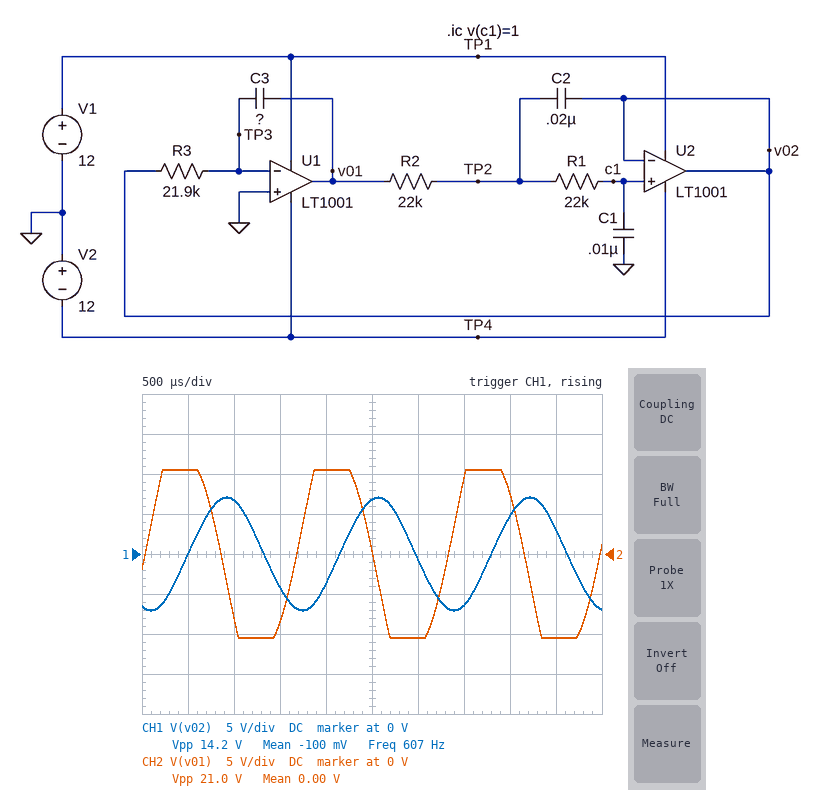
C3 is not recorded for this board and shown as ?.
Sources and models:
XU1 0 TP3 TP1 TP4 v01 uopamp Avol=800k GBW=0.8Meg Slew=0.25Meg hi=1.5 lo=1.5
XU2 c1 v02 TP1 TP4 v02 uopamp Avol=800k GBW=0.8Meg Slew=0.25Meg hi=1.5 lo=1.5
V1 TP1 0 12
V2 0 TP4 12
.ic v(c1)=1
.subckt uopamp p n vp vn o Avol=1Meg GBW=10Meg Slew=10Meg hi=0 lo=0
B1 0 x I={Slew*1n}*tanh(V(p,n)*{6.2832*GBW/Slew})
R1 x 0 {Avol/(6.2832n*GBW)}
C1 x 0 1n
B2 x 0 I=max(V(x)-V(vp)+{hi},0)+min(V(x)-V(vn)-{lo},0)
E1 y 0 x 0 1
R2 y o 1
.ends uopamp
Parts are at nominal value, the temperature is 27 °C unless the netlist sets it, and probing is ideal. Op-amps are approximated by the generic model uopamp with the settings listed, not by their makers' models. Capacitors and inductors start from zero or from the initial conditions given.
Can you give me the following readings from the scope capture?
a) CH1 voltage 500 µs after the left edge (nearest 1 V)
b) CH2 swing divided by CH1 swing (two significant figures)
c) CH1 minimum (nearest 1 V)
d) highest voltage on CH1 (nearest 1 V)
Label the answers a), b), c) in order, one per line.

a) 0 V
b) 1.5
c) -7 V
d) 7 V
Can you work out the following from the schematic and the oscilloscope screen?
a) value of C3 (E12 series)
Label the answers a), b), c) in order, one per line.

a) 5.6 nF
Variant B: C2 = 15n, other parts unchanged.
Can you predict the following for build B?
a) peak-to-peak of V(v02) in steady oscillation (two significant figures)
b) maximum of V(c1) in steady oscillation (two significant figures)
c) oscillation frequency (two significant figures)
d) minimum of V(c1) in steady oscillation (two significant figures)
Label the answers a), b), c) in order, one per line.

a) 13 V
b) 6.4 V
c) 650 Hz
d) -6.4 V
